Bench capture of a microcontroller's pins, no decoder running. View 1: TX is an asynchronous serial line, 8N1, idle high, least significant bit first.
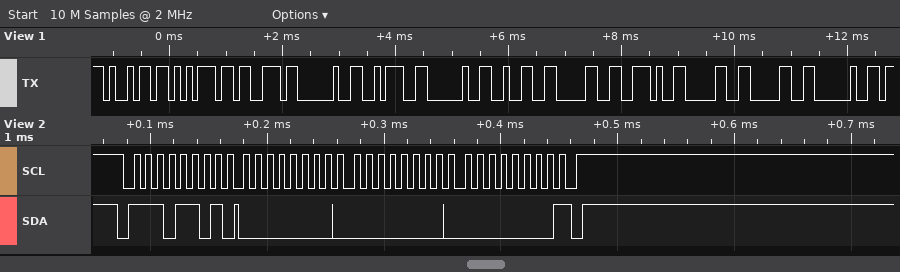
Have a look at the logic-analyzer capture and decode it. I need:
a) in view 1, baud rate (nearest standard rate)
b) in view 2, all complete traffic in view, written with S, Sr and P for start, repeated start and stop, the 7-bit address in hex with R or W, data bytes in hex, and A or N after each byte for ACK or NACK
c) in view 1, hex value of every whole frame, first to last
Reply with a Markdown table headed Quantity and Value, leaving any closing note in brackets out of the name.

| Quantity | Value |
|---|---|
| in view 1, baud rate | 9600 baud |
| in view 2, all complete traffic in view, written with S, Sr and P for start, repeated start and stop, the 7-bit address in hex with R or W, data bytes in hex, and A or N after each byte for ACK or NACK | S 76R A 00 A 00 A 00 N P |
| in view 1, hex value of every whole frame, first to last | 0x69 0x75 0x73 0x20 0x3A 0x20 0x32 0x30 0x2E 0x30 0x30 0x20 |
